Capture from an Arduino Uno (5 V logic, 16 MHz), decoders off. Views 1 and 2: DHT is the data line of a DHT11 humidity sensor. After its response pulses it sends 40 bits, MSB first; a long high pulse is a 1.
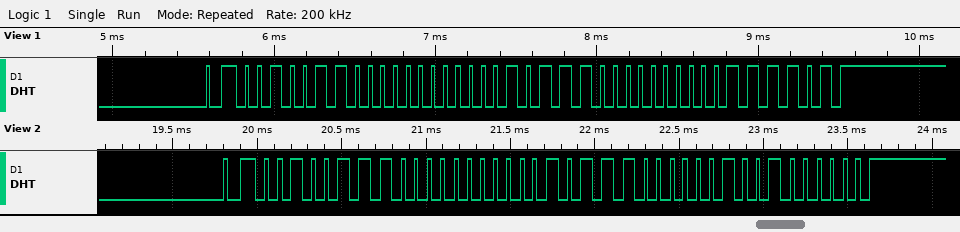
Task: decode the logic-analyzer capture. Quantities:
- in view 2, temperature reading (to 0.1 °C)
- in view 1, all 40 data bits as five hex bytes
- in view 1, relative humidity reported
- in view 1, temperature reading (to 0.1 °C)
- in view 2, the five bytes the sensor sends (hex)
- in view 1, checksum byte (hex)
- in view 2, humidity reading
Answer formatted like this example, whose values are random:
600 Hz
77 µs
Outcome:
23.2 °C
26 00 17 00 3D
38 %
23.0 °C
27 00 17 02 40
0x3D
39 %
